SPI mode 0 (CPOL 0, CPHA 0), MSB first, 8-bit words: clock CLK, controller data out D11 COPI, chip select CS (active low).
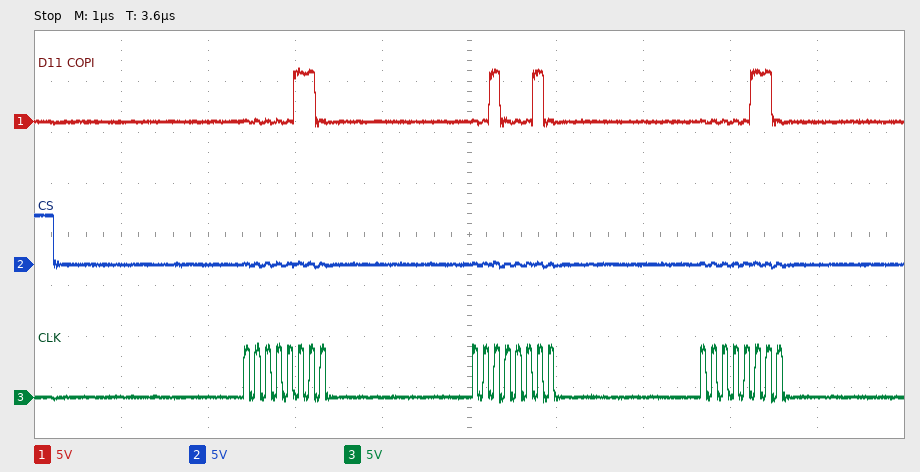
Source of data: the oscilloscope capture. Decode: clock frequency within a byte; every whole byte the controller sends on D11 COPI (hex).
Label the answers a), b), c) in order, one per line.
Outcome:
a) 8 MHz
b) 06 22 06
